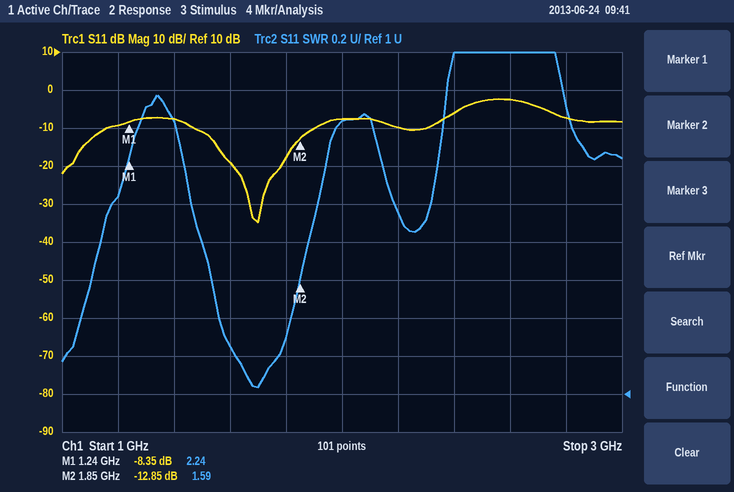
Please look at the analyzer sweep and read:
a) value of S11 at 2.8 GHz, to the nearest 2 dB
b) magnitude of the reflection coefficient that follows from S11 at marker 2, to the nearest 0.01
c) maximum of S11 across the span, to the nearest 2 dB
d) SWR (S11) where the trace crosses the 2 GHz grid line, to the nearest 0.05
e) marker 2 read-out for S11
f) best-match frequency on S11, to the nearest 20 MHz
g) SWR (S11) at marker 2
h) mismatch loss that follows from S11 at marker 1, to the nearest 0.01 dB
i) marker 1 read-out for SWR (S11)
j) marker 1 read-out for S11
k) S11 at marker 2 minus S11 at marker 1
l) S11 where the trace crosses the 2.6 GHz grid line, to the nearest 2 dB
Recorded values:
-8 dB
0.23
-2 dB
2.45
-12.85 dB
1.70 GHz
1.59
0.69 dB
2.24
-8.35 dB
-4.50 dB
-2 dB
